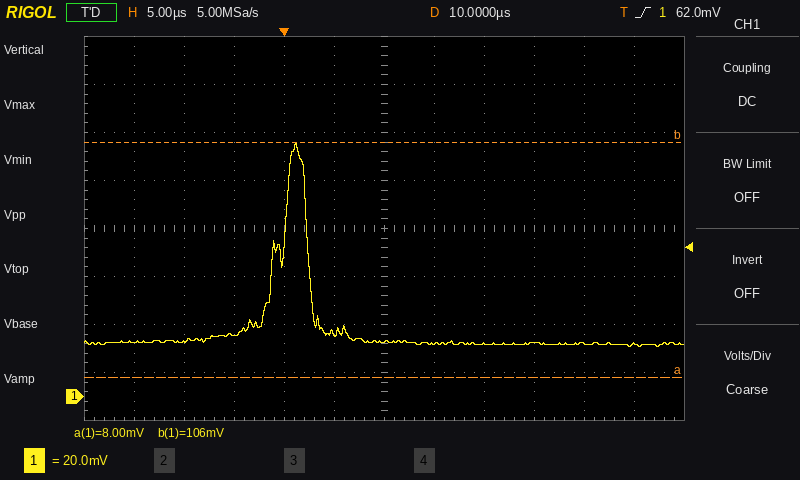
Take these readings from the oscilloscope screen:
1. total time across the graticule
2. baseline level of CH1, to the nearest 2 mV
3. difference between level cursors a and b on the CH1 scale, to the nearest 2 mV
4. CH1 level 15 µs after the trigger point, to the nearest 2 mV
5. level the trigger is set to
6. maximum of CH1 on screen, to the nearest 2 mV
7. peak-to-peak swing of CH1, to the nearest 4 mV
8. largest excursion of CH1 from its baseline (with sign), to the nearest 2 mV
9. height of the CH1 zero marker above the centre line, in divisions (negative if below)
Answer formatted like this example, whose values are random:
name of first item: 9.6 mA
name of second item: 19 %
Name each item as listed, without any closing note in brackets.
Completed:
total time across the graticule: 60 µs
baseline level of CH1, to the nearest 2 mV: 22 mV
difference between level cursors a and b on the CH1 scale, to the nearest 2 mV: 98 mV
CH1 level 15 µs after the trigger point, to the nearest 2 mV: 22 mV
level the trigger is set to: 62.0 mV
maximum of CH1 on screen, to the nearest 2 mV: 106 mV
peak-to-peak swing of CH1, to the nearest 4 mV: 84 mV
largest excursion of CH1 from its baseline (with sign), to the nearest 2 mV: +84 mV
height of the CH1 zero marker above the centre line, in divisions: -3.5 div
